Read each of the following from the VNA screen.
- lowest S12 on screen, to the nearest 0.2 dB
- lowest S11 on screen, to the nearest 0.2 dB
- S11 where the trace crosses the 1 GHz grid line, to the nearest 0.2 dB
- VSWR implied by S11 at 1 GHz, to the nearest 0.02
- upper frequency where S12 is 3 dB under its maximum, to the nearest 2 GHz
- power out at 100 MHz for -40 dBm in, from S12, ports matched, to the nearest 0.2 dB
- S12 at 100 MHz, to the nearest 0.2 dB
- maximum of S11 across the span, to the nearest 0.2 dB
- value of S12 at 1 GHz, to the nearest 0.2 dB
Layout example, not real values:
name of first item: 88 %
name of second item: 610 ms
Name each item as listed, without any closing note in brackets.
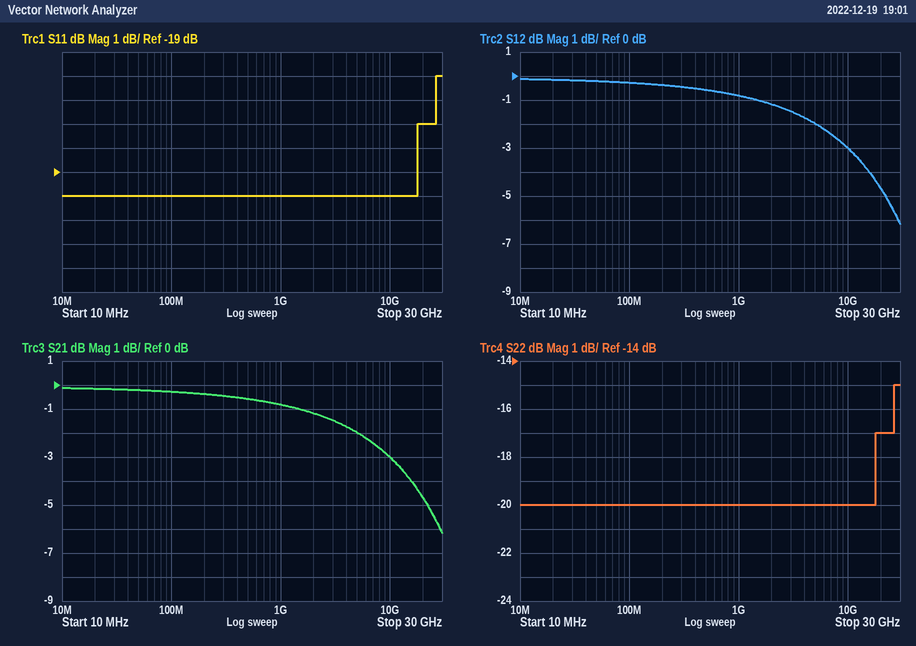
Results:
lowest S12 on screen, to the nearest 0.2 dB: -6.2 dB
lowest S11 on screen, to the nearest 0.2 dB: -20.0 dB
S11 where the trace crosses the 1 GHz grid line, to the nearest 0.2 dB: -20.0 dB
VSWR implied by S11 at 1 GHz, to the nearest 0.02: 1.22
upper frequency where S12 is 3 dB under its maximum, to the nearest 2 GHz: 10 GHz
power out at 100 MHz for -40 dBm in, from S12, ports matched, to the nearest 0.2 dB: -40.2 dBm
S12 at 100 MHz, to the nearest 0.2 dB: -0.2 dB
maximum of S11 across the span, to the nearest 0.2 dB: -15.0 dB
value of S12 at 1 GHz, to the nearest 0.2 dB: -0.8 dB
